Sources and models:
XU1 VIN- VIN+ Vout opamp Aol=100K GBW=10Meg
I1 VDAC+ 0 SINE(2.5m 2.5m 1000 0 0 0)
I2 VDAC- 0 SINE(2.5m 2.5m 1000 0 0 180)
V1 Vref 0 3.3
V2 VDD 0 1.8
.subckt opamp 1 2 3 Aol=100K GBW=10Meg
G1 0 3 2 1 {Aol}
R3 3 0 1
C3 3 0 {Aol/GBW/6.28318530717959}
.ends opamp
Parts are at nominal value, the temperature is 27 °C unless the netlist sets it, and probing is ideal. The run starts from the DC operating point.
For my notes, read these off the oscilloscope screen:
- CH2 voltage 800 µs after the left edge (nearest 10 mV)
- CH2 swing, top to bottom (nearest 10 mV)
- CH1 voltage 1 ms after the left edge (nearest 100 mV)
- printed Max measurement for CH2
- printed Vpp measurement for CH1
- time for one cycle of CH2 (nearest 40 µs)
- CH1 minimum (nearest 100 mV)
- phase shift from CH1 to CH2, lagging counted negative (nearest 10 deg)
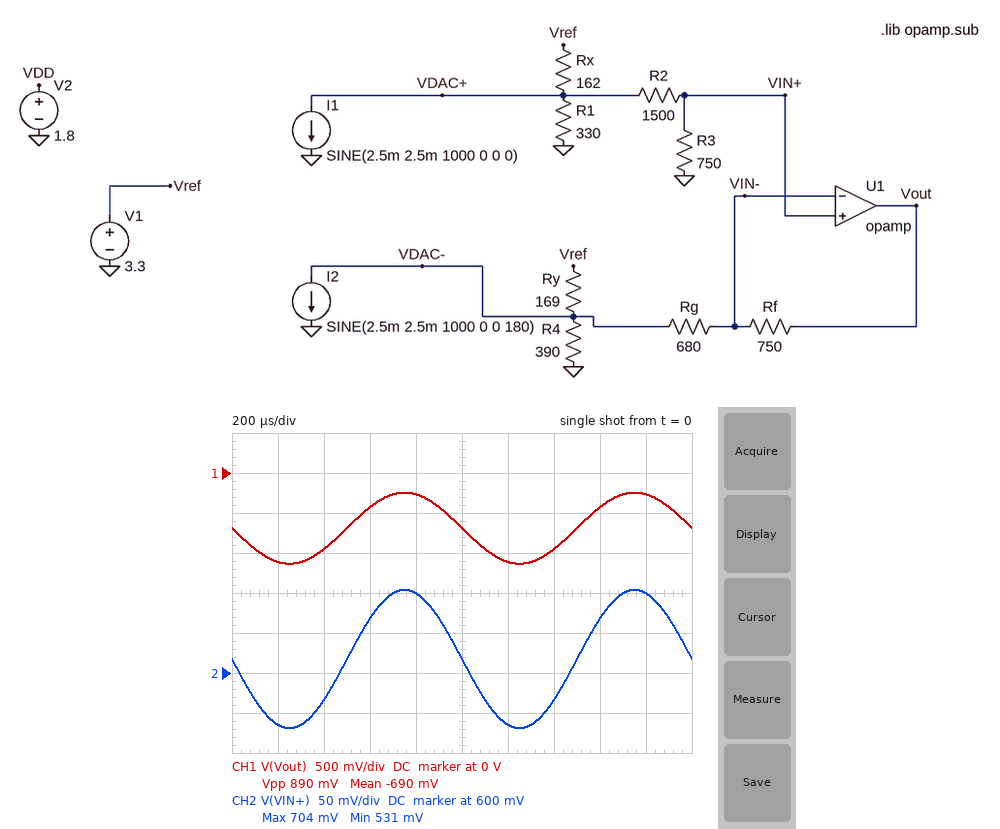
700 mV
170 mV
-700 mV
704 mV
890 mV
1.00 ms
-1.1 V
0 deg
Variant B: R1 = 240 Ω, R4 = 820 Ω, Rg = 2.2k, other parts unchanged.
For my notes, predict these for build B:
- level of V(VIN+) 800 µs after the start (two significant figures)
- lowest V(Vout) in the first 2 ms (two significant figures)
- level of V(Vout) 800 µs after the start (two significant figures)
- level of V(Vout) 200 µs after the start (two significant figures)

630 mV
-250 mV
170 mV
-240 mV
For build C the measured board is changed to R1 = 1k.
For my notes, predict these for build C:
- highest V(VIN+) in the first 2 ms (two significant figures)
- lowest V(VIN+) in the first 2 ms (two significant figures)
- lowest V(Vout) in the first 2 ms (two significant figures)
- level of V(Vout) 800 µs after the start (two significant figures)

890 mV
670 mV
-860 mV
95 mV
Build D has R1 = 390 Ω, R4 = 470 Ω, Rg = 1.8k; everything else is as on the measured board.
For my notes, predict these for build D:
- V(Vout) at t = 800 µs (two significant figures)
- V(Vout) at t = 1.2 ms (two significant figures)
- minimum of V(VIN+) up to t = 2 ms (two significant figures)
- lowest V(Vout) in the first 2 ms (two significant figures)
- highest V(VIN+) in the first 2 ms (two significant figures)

310 mV
-160 mV
560 mV
-170 mV
740 mV
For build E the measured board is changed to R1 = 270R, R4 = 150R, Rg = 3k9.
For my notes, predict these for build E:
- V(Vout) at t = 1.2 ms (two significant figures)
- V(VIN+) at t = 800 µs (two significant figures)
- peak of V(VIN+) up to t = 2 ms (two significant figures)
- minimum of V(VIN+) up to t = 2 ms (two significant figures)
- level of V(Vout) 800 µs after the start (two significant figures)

300 mV
650 mV
660 mV
500 mV
560 mV
